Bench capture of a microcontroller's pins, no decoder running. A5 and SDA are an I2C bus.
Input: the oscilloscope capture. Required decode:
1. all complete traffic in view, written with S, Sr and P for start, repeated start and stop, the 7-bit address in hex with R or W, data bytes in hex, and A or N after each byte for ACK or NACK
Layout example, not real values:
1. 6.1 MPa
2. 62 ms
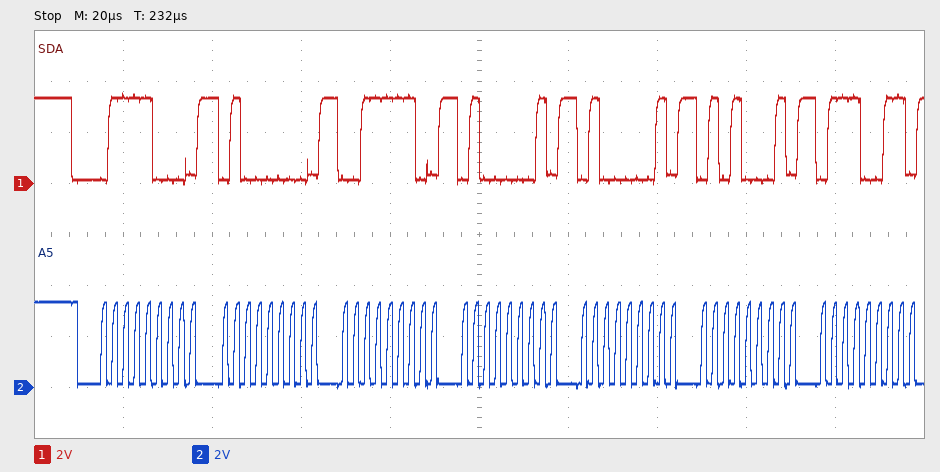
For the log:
1. S 3CW A 40 A 3E A 41 A 41 A 51 A 73 A
